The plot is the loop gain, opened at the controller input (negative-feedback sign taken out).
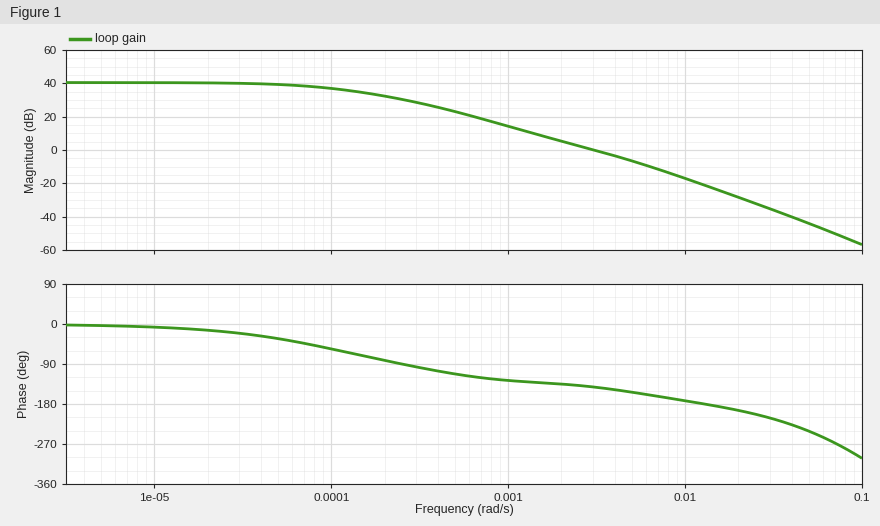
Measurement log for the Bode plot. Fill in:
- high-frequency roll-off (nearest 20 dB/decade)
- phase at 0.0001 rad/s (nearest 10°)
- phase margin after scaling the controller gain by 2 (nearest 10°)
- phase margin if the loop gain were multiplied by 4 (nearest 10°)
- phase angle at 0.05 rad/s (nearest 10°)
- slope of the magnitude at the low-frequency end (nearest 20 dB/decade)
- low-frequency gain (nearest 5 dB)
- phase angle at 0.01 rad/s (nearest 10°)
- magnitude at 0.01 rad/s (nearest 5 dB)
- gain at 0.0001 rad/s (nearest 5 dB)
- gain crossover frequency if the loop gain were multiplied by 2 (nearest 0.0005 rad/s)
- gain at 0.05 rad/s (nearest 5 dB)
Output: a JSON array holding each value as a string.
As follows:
["-40 dB/decade", "-60°", "30°", "20°", "-240°", "0 dB/decade", "40 dB", "-170°", "-15 dB", "35 dB", "0.0050 rad/s", "-45 dB"]
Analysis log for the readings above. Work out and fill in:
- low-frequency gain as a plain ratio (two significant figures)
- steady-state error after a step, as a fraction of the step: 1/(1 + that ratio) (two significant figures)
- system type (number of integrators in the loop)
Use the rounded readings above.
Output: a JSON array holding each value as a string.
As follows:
["100", "0.0099", "0"]
